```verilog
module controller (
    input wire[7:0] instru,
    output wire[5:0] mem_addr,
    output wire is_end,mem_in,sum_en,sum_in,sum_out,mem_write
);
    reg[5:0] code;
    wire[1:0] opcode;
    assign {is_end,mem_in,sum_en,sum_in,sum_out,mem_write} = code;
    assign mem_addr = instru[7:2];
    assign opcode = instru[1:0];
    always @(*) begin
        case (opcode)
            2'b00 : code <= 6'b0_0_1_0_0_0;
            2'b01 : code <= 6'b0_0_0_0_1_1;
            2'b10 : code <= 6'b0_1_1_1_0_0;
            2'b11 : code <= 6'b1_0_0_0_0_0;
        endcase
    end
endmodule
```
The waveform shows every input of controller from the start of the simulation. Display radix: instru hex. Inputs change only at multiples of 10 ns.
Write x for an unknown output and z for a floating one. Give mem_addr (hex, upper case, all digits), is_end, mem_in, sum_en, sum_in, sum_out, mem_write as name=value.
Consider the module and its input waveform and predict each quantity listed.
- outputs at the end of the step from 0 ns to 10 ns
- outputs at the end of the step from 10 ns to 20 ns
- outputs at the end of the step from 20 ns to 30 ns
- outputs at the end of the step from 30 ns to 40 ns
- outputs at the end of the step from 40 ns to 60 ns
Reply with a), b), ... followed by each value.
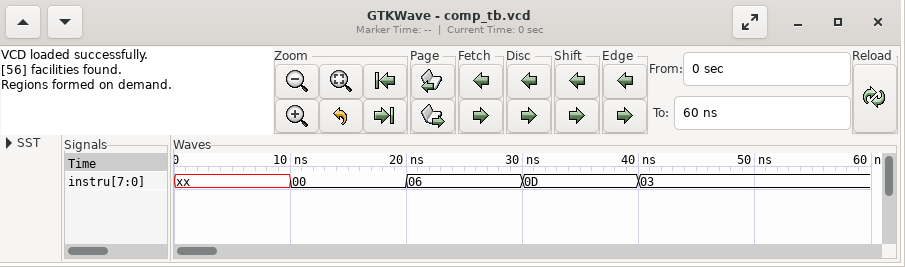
a) mem_addr=x, is_end=x, mem_in=x, sum_en=x, sum_in=x, sum_out=x, mem_write=x
b) mem_addr=00, is_end=0, mem_in=0, sum_en=1, sum_in=0, sum_out=0, mem_write=0
c) mem_addr=01, is_end=0, mem_in=1, sum_en=1, sum_in=1, sum_out=0, mem_write=0
d) mem_addr=03, is_end=0, mem_in=0, sum_en=0, sum_in=0, sum_out=1, mem_write=1
e) mem_addr=00, is_end=1, mem_in=0, sum_en=0, sum_in=0, sum_out=0, mem_write=0
